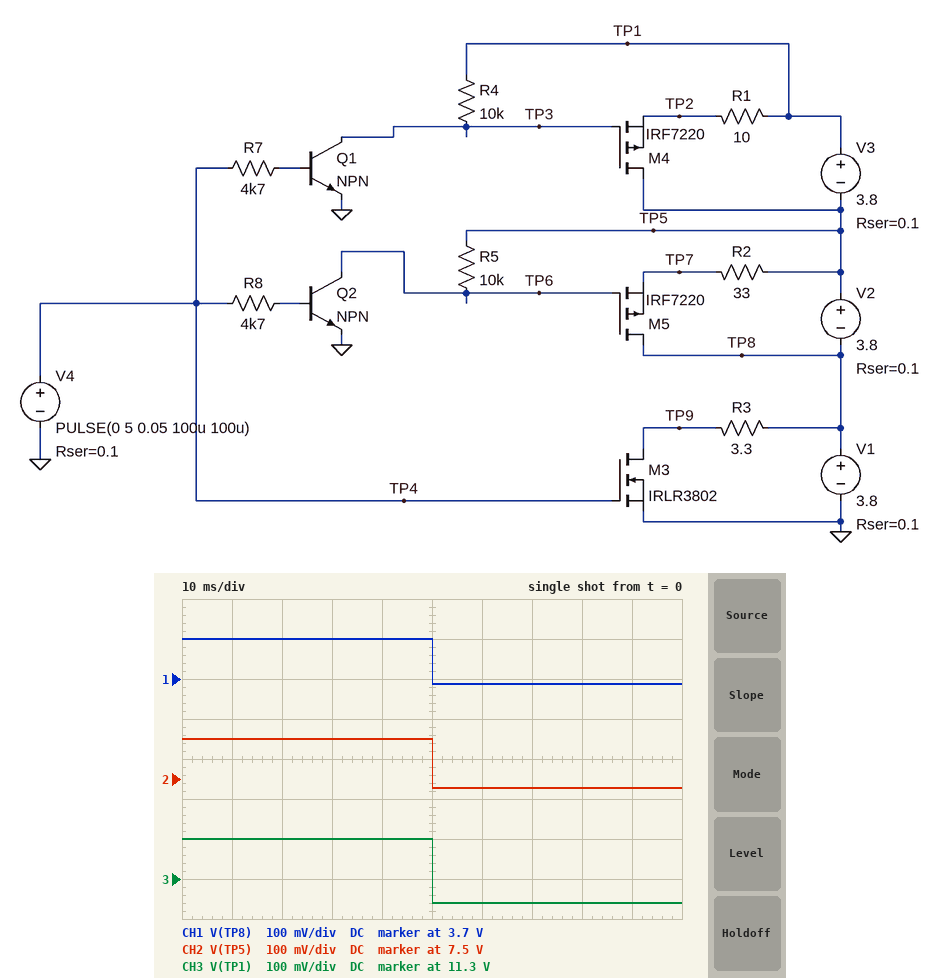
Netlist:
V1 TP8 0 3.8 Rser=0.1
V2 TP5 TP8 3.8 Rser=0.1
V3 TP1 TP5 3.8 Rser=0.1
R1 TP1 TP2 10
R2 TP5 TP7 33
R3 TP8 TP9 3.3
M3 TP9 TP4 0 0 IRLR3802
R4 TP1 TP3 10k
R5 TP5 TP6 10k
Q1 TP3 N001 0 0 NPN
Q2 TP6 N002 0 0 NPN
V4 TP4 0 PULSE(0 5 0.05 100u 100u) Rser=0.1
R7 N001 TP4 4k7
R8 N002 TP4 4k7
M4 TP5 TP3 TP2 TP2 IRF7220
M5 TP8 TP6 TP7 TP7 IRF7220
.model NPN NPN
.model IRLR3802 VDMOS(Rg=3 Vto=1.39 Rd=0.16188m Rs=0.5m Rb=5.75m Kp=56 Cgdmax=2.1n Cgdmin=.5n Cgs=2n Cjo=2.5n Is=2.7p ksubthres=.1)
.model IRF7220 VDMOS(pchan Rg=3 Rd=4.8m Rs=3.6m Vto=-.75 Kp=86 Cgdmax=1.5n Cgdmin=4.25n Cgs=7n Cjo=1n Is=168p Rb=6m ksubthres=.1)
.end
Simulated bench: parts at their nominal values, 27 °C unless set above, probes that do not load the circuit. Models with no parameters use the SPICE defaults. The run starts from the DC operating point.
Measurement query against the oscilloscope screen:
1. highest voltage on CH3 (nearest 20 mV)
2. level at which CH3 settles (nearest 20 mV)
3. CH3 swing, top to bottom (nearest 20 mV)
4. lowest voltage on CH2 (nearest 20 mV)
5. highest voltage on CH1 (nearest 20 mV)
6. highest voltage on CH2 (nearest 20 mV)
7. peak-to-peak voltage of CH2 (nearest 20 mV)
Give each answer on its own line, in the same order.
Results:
11.40 V
11.24 V
160 mV
7.48 V
3.80 V
7.60 V
120 mV
